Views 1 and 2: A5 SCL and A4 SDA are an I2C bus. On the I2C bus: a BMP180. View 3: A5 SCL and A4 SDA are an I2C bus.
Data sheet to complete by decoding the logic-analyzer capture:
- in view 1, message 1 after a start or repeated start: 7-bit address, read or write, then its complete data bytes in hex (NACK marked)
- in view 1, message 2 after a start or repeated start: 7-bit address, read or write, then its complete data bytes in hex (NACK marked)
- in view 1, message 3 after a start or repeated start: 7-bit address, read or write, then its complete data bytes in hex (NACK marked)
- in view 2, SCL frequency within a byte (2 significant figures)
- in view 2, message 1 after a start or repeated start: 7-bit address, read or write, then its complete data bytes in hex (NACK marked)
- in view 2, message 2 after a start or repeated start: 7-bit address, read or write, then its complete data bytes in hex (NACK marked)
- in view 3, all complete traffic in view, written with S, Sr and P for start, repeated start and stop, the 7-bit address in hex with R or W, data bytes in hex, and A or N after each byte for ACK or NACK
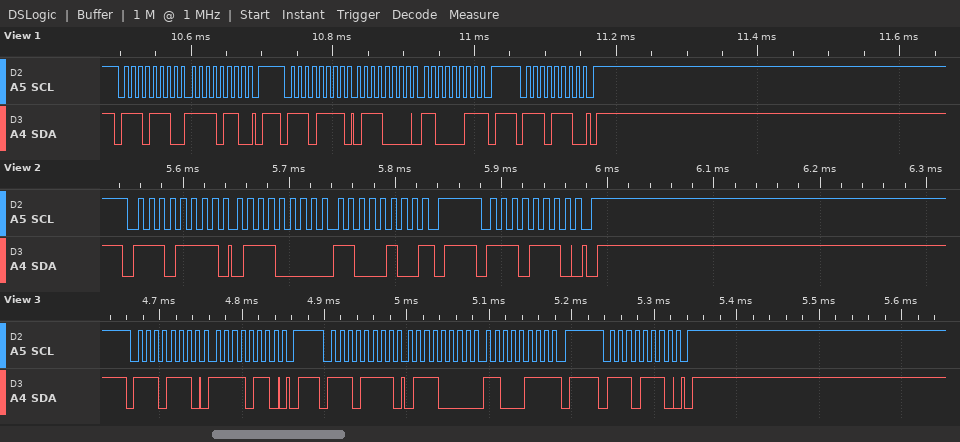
0x77 write: F6
0x77 read: 70 C3 NACK
0x77 write
100 kHz
0x77 read: 70 C4 NACK
0x77 write
S 77W A F6 A P S 77R A 70 A C7 N P S 77W A P
